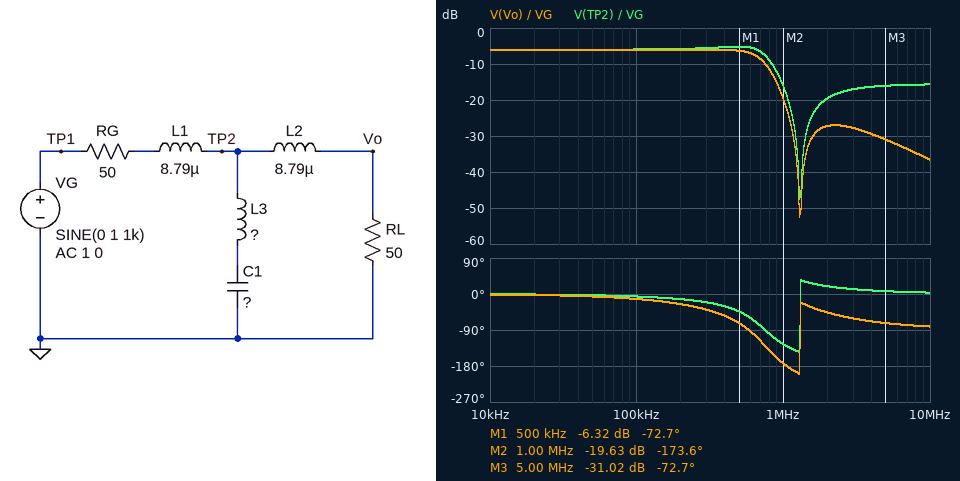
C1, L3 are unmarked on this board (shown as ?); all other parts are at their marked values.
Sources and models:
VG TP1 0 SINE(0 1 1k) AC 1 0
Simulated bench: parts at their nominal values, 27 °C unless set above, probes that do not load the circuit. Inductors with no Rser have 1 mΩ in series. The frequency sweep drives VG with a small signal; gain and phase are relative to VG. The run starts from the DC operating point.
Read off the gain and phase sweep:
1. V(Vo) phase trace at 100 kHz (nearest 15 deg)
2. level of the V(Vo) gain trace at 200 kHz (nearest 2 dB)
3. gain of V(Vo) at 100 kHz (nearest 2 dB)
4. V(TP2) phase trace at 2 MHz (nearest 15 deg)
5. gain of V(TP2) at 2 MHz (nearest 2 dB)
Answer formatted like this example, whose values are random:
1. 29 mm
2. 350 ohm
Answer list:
1. -15 deg
2. -6 dB
3. -6 dB
4. 15 deg
5. -20 dB
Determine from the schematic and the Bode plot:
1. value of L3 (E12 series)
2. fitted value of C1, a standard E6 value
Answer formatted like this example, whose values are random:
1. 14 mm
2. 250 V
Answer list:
1. 2.2 µH
2. 6.8 nF
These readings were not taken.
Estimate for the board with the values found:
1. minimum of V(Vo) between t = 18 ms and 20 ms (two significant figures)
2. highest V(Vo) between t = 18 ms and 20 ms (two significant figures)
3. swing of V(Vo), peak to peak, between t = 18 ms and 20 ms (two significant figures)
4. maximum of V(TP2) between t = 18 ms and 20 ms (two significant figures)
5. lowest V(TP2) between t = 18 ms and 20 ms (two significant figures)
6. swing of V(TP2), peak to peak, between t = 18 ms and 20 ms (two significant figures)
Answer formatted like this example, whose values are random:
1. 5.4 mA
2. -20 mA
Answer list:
1. -500 mV
2. 500 mV
3. 1.0 V
4. 500 mV
5. -500 mV
6. 1.0 V
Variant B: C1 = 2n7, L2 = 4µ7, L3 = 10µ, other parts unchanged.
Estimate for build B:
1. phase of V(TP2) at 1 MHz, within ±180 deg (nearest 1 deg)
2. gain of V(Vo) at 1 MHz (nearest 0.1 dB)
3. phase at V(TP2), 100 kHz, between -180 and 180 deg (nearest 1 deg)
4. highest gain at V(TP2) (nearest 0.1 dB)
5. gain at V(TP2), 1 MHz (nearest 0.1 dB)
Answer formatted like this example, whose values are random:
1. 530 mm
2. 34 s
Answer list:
1. 37 deg
2. -27.6 dB
3. -4 deg
4. -5.6 dB
5. -26.3 dB
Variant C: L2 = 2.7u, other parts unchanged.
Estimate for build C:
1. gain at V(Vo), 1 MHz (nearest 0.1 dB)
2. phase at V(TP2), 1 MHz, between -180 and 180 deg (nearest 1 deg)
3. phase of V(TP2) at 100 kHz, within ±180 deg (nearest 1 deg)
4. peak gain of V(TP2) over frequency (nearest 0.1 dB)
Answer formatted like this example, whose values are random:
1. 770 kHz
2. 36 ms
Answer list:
1. -17.2 dB
2. -121 deg
3. -8 deg
4. -6.0 dB
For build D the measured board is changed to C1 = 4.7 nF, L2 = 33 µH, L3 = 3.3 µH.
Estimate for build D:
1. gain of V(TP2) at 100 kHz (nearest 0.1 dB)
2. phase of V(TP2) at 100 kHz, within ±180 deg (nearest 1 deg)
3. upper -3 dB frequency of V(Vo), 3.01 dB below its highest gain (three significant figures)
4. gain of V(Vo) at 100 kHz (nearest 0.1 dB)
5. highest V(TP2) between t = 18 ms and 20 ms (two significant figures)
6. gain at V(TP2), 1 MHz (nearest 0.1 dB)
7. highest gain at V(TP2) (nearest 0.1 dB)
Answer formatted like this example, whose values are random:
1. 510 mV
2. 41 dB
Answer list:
1. -5.5 dB
2. 3 deg
3. 590 kHz
4. -6.2 dB
5. 500 mV
6. -13.4 dB
7. -0.5 dB
